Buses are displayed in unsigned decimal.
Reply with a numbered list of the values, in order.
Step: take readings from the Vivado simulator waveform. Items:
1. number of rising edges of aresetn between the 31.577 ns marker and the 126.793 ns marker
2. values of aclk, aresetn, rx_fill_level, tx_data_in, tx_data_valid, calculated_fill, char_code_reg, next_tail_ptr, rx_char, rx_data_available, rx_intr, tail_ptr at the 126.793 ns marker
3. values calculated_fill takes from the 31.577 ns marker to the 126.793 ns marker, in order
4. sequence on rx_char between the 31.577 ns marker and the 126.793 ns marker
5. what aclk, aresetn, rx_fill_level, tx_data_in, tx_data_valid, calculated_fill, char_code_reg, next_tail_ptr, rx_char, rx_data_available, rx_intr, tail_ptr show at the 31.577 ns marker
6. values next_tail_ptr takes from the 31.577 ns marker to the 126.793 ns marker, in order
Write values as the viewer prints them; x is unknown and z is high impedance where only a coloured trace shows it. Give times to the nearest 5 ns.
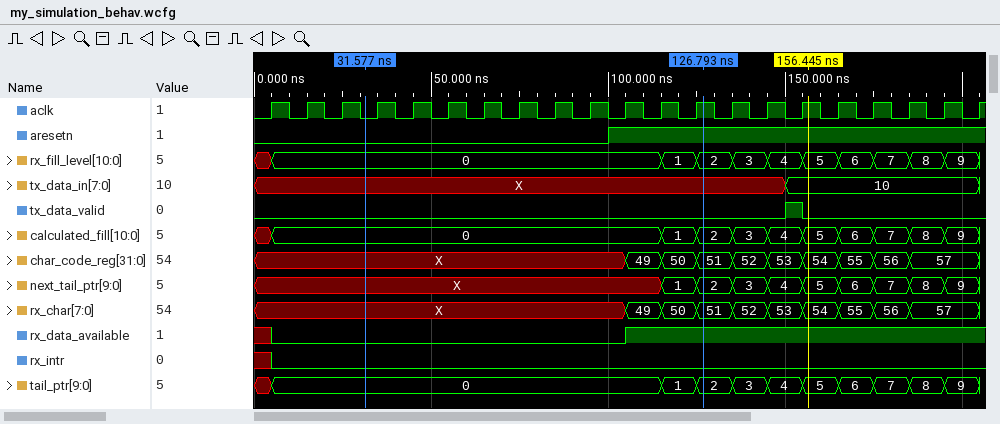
1. 1
2. aclk=1, aresetn=1, rx_fill_level=2, tx_data_in=X, tx_data_valid=0, calculated_fill=2, char_code_reg=51, next_tail_ptr=2, rx_char=51, rx_data_available=1, rx_intr=0, tail_ptr=2
3. 0, 1, 2
4. X, 49, 50, 51
5. aclk=0, aresetn=0, rx_fill_level=0, tx_data_in=X, tx_data_valid=0, calculated_fill=0, char_code_reg=X, next_tail_ptr=X, rx_char=X, rx_data_available=0, rx_intr=0, tail_ptr=0
6. X, 1, 2
